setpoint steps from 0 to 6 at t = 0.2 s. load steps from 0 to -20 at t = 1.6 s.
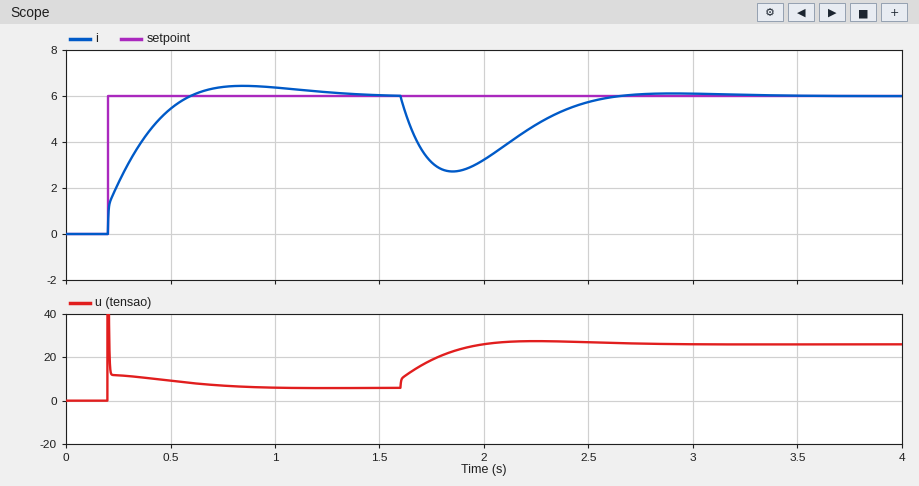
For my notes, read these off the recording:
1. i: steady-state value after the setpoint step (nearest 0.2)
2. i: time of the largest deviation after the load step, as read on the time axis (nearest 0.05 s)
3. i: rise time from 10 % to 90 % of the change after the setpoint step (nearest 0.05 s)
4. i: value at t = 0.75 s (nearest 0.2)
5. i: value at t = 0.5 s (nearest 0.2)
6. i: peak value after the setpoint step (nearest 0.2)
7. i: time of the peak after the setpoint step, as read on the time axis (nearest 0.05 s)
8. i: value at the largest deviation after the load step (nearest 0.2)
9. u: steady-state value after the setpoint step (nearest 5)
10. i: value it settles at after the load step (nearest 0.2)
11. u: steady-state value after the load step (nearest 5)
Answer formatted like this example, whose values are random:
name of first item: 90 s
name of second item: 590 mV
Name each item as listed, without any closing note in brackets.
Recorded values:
i: steady-state value after the setpoint step: 6.0
i: time of the largest deviation after the load step, as read on the time axis: 1.85 s
i: rise time from 10 % to 90 % of the change after the setpoint step: 0.30 s
i: value at t = 0.75 s: 6.4
i: value at t = 0.5 s: 5.4
i: peak value after the setpoint step: 6.4
i: time of the peak after the setpoint step, as read on the time axis: 0.85 s
i: value at the largest deviation after the load step: 2.8
u: steady-state value after the setpoint step: 5
i: value it settles at after the load step: 6.0
u: steady-state value after the load step: 25
